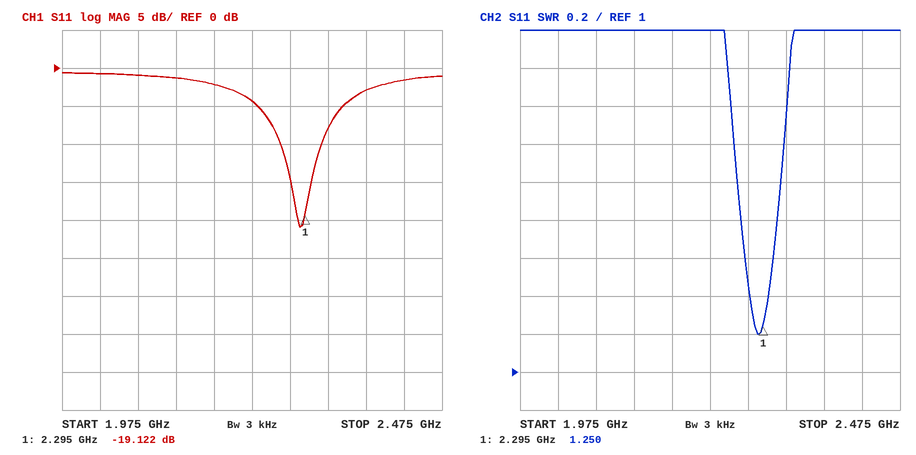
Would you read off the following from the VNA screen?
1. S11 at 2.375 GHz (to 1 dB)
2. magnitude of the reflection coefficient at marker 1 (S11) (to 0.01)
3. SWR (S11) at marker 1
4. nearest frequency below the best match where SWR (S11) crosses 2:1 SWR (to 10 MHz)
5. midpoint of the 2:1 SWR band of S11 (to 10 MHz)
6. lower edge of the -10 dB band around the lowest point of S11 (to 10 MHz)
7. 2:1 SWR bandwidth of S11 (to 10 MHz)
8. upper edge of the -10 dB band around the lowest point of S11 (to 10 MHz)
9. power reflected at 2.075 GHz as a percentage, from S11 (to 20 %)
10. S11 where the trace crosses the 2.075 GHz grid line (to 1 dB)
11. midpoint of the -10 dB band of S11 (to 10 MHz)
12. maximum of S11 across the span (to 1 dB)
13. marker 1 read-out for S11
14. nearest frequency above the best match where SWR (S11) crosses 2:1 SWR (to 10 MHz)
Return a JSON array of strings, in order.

["-3 dB", "0.11", "1.250", "2.26 GHz", "2.29 GHz", "2.26 GHz", "60 MHz", "2.32 GHz", "80 %", "-1 dB", "2.29 GHz", "-1 dB", "-19.122 dB", "2.32 GHz"]
